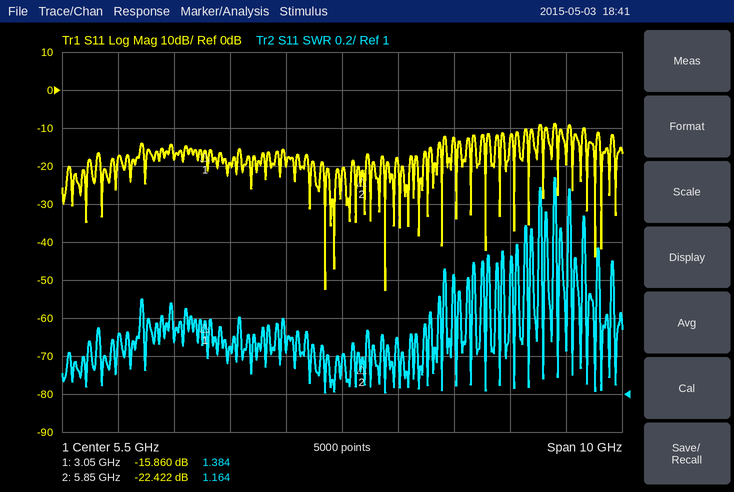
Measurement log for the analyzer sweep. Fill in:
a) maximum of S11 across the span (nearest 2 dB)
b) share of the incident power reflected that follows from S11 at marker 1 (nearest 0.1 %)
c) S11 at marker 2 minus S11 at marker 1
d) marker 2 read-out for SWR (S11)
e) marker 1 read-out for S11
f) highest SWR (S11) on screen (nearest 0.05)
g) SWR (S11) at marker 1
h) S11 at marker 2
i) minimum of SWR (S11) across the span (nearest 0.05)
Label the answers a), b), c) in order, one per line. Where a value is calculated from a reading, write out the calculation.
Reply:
a) -8 dB
b) 10^(-15.86/10) ≈ 2.6 %
c) -22.422 − (-15.86) = -6.562 dB
d) 1.164
e) -15.860 dB
f) 2.15
g) 1.384
h) -22.422 dB
i) 1.00
